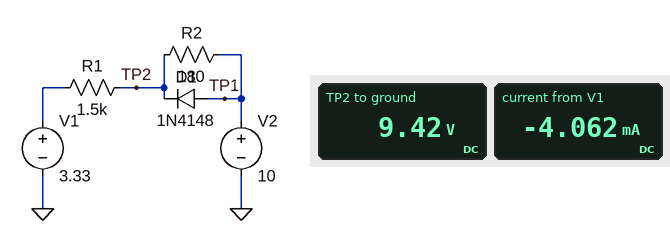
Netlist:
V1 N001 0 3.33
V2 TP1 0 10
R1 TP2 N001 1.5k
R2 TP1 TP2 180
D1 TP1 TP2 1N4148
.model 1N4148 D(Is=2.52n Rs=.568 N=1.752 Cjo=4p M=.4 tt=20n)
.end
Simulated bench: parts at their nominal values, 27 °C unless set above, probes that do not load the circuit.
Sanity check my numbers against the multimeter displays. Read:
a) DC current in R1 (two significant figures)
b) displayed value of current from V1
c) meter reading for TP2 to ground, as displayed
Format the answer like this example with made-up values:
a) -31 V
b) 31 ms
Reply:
a) 4.1 mA
b) -4.062 mA
c) 9.42 V
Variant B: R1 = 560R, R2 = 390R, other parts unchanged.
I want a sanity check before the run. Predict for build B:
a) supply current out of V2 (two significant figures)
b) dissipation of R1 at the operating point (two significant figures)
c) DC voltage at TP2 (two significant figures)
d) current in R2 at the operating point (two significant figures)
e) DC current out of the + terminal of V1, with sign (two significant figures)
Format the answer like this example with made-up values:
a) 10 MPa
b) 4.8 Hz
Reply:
a) 11 mA
b) 64 mW
c) 9.3 V
d) 1.8 mA
e) -11 mA
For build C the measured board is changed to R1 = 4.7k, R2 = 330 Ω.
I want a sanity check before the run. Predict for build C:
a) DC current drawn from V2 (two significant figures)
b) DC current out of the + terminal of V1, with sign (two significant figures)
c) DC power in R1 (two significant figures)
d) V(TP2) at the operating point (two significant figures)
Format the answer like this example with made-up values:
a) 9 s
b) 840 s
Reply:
a) 1.3 mA
b) -1.3 mA
c) 8.3 mW
d) 9.6 V
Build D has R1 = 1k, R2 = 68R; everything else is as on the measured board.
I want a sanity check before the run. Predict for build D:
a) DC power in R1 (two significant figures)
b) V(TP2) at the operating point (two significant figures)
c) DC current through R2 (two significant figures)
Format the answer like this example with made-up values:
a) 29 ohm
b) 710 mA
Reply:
a) 39 mW
b) 9.6 V
c) 6.2 mA
